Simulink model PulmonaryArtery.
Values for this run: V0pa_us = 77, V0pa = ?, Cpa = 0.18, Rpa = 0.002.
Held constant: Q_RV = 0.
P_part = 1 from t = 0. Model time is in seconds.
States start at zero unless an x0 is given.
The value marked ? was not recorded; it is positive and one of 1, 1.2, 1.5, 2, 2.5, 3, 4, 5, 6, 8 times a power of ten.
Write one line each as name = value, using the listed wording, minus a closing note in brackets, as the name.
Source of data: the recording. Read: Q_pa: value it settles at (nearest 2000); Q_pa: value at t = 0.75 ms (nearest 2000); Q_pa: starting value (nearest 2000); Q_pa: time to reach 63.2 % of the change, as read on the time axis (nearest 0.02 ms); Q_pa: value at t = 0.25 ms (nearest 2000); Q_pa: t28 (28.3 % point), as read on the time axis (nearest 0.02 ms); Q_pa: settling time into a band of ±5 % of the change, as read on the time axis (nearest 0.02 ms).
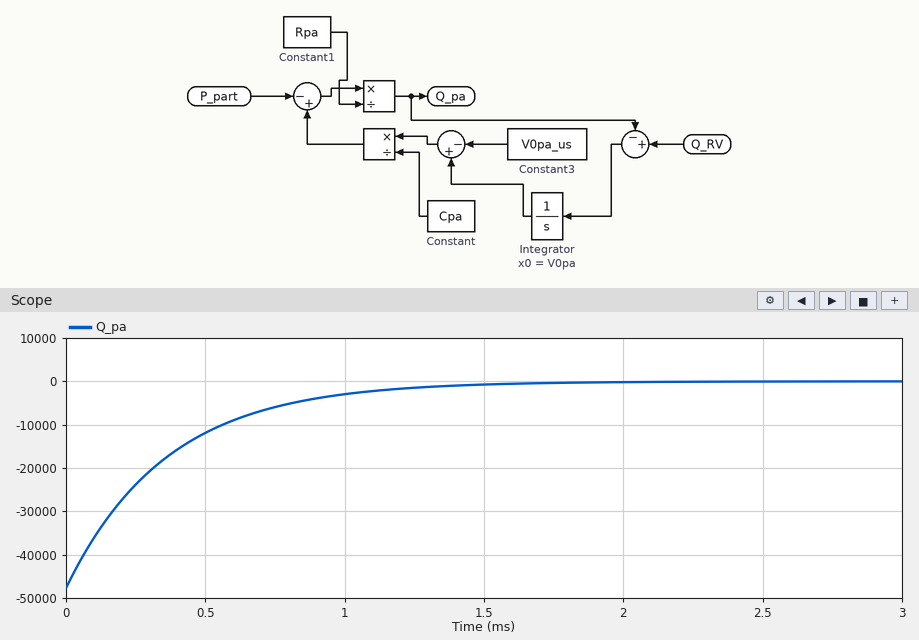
Q_pa: value it settles at = 0
Q_pa: value at t = 0.75 ms = -6000
Q_pa: starting value = -48000
Q_pa: time to reach 63.2 % of the change, as read on the time axis = 0.36 ms
Q_pa: value at t = 0.25 ms = -24000
Q_pa: t28 (28.3 % point), as read on the time axis = 0.12 ms
Q_pa: settling time into a band of ±5 % of the change, as read on the time axis = 1.08 ms
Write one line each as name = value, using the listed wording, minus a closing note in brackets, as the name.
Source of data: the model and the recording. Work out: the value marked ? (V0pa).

the value marked ? = 60
